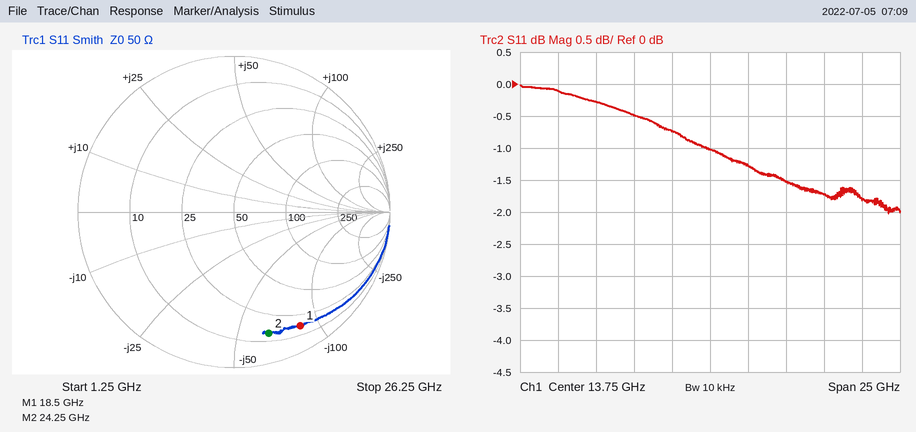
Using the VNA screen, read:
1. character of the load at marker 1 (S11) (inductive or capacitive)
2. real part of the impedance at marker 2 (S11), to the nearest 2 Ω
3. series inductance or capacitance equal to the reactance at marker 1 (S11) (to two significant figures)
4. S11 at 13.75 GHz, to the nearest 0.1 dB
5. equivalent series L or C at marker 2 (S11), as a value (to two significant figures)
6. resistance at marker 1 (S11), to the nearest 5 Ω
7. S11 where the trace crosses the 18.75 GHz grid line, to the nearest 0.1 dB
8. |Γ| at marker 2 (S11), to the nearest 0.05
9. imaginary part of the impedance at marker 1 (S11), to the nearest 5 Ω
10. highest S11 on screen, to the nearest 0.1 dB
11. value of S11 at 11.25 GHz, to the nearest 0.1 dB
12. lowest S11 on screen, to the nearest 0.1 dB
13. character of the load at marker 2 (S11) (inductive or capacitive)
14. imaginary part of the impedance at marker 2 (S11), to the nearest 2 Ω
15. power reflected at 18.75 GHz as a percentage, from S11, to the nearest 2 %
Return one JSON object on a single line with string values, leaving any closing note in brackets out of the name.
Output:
{"character of the load at marker 1 (S11)": "capacitive", "real part of the impedance at marker 2 (S11), to the nearest 2 Ω": "14 Ω", "series inductance or capacitance equal to the reactance at marker 1 (S11)": "100 fF", "S11 at 13.75 GHz, to the nearest 0.1 dB": "-1.0 dB", "equivalent series L or C at marker 2 (S11), as a value": "100 fF", "resistance at marker 1 (S11), to the nearest 5 Ω": "15 Ω", "S11 where the trace crosses the 18.75 GHz grid line, to the nearest 0.1 dB": "-1.5 dB", "|Γ| at marker 2 (S11), to the nearest 0.05": "0.80", "imaginary part of the impedance at marker 1 (S11), to the nearest 5 Ω": "-85 Ω", "highest S11 on screen, to the nearest 0.1 dB": "0.0 dB", "value of S11 at 11.25 GHz, to the nearest 0.1 dB": "-0.7 dB", "lowest S11 on screen, to the nearest 0.1 dB": "-2.0 dB", "character of the load at marker 2 (S11)": "capacitive", "imaginary part of the impedance at marker 2 (S11), to the nearest 2 Ω": "-64 Ω", "power reflected at 18.75 GHz as a percentage, from S11, to the nearest 2 %": "70 %"}
